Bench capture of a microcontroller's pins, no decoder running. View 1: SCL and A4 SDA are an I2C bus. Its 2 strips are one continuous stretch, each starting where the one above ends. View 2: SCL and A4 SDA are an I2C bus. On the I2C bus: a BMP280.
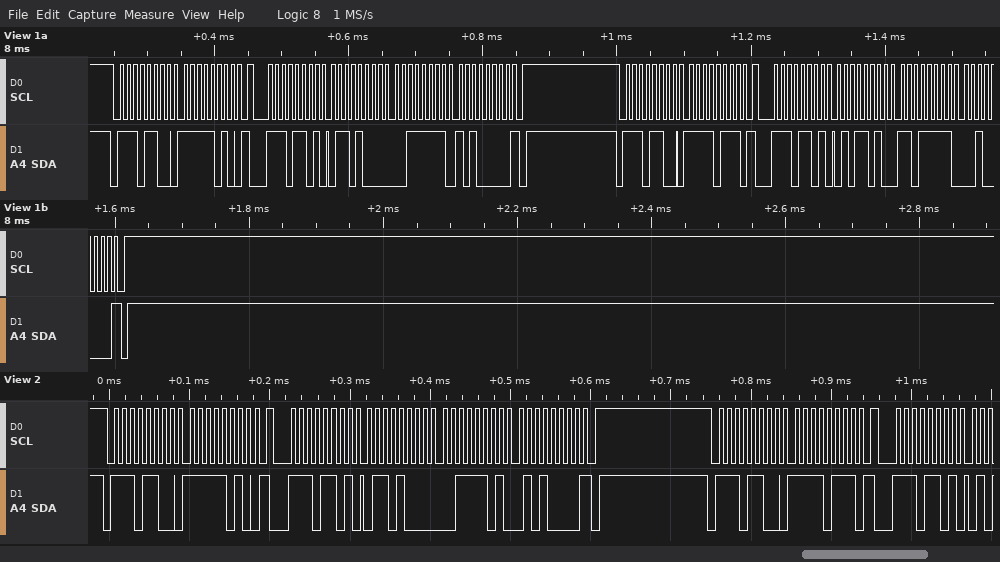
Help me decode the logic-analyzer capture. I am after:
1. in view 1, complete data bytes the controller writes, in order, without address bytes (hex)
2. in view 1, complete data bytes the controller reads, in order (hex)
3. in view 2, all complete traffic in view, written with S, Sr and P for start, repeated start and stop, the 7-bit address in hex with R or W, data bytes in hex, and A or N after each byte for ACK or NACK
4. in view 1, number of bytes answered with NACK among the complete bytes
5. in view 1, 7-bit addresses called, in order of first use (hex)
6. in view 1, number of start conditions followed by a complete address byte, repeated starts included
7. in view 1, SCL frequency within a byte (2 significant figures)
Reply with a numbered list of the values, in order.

1. FA F7
2. 68 3F A0 5A DF 20
3. S 76W A FA A Sr 76R A 68 A 3D A 50 N P S 76W A F7 A Sr 76R A
4. 2
5. 0x76
6. 4
7. 100 kHz
